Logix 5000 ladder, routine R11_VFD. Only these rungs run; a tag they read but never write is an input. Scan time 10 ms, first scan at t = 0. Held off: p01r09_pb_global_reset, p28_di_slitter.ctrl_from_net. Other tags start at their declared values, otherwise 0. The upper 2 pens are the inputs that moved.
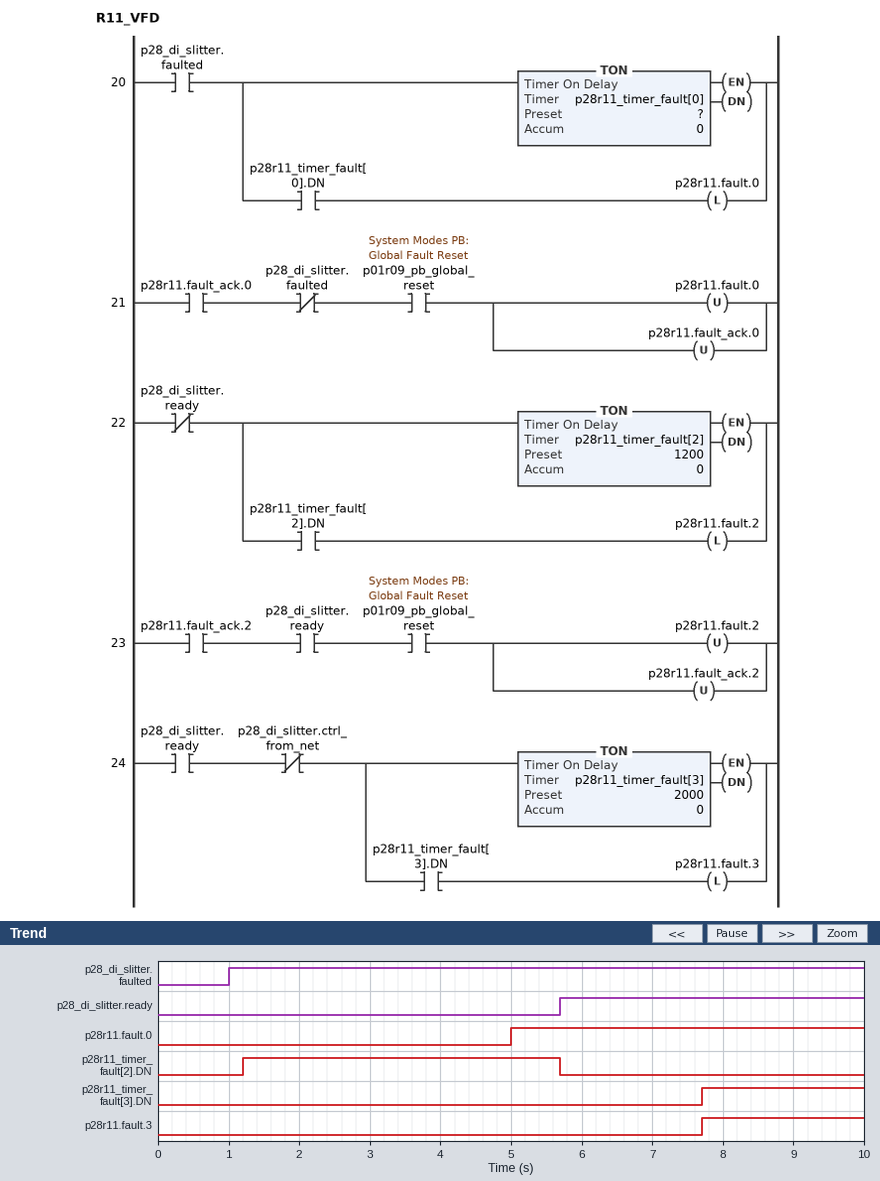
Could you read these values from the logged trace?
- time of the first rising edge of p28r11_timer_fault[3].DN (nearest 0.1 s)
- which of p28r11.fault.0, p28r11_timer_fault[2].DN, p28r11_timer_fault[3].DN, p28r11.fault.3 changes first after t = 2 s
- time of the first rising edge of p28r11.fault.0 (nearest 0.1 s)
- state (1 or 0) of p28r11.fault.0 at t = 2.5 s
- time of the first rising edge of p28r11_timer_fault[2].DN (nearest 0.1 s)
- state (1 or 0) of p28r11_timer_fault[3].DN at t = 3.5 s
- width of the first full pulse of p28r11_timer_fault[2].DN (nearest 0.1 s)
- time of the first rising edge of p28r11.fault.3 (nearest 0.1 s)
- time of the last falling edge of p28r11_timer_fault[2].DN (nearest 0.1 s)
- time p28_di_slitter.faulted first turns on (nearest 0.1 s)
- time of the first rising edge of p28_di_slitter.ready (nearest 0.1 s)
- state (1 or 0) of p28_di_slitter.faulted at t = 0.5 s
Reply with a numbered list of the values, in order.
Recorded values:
1. 7.7 s
2. p28r11.fault.0
3. 5.0 s
4. 0
5. 1.2 s
6. 0
7. 4.5 s
8. 7.7 s
9. 5.7 s
10. 1.0 s
11. 5.7 s
12. 0
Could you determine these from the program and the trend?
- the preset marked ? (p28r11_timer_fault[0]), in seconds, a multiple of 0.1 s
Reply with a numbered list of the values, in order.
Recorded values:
1. 4.0 s
